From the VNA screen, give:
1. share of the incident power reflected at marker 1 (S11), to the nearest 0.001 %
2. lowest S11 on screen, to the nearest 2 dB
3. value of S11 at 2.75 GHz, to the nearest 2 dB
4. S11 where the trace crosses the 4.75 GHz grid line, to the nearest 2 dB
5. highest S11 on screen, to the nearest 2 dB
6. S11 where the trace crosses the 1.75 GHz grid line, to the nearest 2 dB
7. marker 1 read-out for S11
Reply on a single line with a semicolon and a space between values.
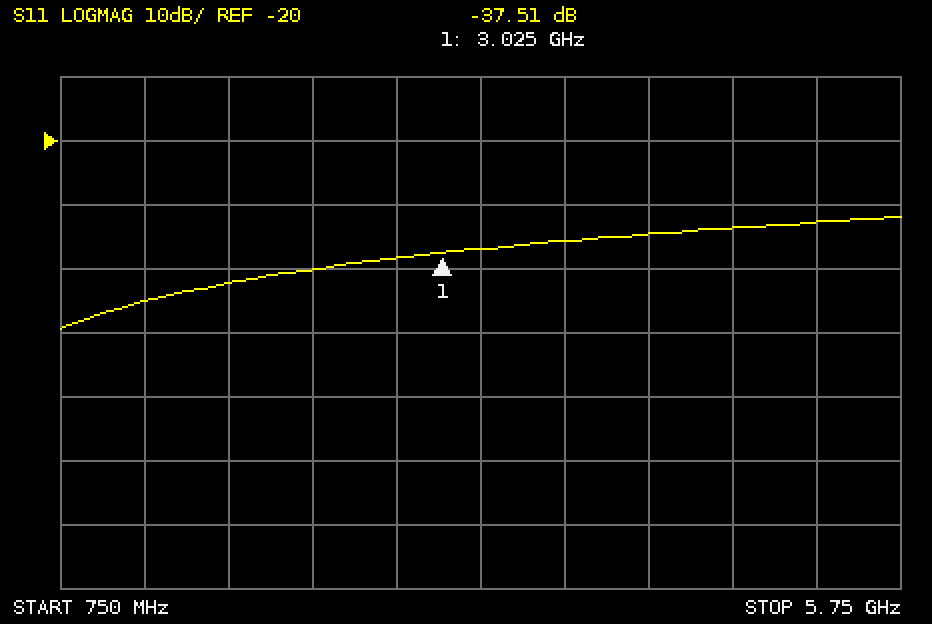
0.018 %; -50 dB; -38 dB; -34 dB; -32 dB; -42 dB; -37.51 dB
